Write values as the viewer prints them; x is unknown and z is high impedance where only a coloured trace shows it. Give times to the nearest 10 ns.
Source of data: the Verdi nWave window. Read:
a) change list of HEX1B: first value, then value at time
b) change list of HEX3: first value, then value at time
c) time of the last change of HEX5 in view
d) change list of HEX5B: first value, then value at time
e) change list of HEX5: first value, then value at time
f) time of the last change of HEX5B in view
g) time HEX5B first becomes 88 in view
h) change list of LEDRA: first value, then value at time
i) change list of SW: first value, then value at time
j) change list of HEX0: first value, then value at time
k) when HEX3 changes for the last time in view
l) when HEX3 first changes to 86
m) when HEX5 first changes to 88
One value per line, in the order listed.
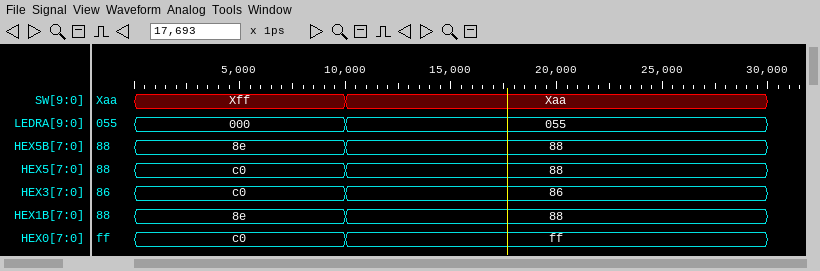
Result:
8e, 88 at 10 ns
c0, 86 at 10 ns
10 ns
8e, 88 at 10 ns
c0, 88 at 10 ns
10 ns
10 ns
000, 055 at 10 ns
Xff, Xaa at 10 ns
c0, ff at 10 ns
10 ns
10 ns
10 ns
